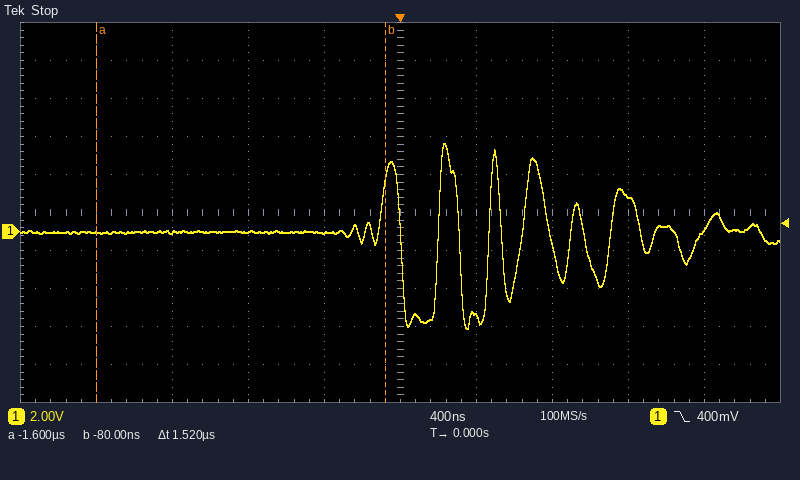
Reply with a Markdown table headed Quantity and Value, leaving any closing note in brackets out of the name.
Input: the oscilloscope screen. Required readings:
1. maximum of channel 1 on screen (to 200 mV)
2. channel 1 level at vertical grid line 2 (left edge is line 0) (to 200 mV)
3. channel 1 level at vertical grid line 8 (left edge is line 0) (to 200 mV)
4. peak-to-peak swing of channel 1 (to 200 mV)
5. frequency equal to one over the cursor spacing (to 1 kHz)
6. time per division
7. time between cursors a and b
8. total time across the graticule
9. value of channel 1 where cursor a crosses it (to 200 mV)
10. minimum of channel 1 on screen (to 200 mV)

| Quantity | Value |
|---|---|
| maximum of channel 1 on screen | 4.6 V |
| channel 1 level at vertical grid line 2 (left edge is line 0) | 0.0 V |
| channel 1 level at vertical grid line 8 (left edge is line 0) | 1.8 V |
| peak-to-peak swing of channel 1 | 9.8 V |
| frequency equal to one over the cursor spacing | 658 kHz |
| time per division | 400 ns |
| time between cursors a and b | 1.52 µs |
| total time across the graticule | 4 µs |
| value of channel 1 where cursor a crosses it | 0.0 V |
| minimum of channel 1 on screen | -5.2 V |
